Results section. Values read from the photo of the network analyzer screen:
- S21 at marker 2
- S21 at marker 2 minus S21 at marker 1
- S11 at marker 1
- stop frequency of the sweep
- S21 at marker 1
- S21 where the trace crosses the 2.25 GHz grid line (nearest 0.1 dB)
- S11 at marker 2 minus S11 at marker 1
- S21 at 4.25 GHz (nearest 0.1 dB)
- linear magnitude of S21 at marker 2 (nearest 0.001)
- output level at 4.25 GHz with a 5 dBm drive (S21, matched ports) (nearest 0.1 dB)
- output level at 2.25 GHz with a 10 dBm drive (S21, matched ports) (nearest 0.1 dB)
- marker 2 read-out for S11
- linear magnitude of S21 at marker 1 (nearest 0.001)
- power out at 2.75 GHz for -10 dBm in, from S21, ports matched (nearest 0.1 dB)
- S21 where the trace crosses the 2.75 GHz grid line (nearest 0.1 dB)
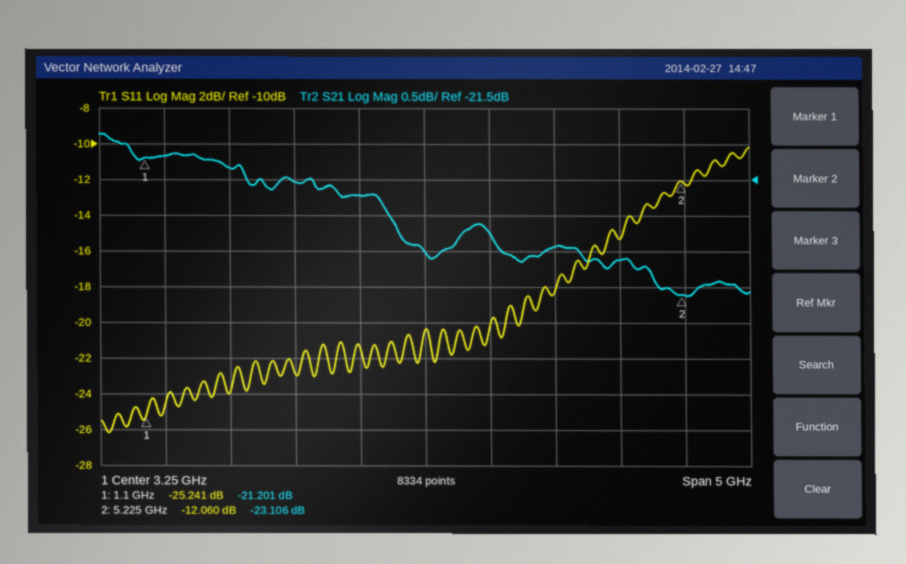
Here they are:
-23.106 dB
-1.905 dB
-25.241 dB
5.75 GHz
-21.201 dB
-21.5 dB
13.181 dB
-22.4 dB
0.070
-17.4 dBm
-11.5 dBm
-12.060 dB
0.087
-31.7 dBm
-21.7 dB
